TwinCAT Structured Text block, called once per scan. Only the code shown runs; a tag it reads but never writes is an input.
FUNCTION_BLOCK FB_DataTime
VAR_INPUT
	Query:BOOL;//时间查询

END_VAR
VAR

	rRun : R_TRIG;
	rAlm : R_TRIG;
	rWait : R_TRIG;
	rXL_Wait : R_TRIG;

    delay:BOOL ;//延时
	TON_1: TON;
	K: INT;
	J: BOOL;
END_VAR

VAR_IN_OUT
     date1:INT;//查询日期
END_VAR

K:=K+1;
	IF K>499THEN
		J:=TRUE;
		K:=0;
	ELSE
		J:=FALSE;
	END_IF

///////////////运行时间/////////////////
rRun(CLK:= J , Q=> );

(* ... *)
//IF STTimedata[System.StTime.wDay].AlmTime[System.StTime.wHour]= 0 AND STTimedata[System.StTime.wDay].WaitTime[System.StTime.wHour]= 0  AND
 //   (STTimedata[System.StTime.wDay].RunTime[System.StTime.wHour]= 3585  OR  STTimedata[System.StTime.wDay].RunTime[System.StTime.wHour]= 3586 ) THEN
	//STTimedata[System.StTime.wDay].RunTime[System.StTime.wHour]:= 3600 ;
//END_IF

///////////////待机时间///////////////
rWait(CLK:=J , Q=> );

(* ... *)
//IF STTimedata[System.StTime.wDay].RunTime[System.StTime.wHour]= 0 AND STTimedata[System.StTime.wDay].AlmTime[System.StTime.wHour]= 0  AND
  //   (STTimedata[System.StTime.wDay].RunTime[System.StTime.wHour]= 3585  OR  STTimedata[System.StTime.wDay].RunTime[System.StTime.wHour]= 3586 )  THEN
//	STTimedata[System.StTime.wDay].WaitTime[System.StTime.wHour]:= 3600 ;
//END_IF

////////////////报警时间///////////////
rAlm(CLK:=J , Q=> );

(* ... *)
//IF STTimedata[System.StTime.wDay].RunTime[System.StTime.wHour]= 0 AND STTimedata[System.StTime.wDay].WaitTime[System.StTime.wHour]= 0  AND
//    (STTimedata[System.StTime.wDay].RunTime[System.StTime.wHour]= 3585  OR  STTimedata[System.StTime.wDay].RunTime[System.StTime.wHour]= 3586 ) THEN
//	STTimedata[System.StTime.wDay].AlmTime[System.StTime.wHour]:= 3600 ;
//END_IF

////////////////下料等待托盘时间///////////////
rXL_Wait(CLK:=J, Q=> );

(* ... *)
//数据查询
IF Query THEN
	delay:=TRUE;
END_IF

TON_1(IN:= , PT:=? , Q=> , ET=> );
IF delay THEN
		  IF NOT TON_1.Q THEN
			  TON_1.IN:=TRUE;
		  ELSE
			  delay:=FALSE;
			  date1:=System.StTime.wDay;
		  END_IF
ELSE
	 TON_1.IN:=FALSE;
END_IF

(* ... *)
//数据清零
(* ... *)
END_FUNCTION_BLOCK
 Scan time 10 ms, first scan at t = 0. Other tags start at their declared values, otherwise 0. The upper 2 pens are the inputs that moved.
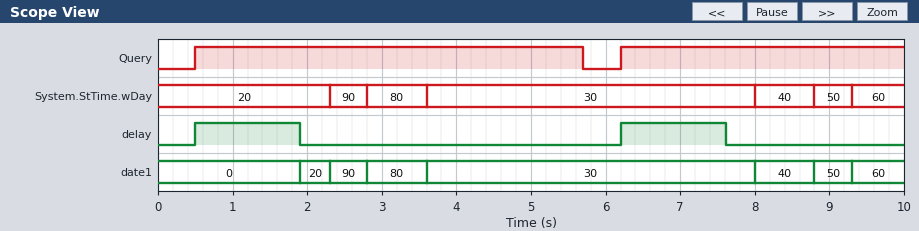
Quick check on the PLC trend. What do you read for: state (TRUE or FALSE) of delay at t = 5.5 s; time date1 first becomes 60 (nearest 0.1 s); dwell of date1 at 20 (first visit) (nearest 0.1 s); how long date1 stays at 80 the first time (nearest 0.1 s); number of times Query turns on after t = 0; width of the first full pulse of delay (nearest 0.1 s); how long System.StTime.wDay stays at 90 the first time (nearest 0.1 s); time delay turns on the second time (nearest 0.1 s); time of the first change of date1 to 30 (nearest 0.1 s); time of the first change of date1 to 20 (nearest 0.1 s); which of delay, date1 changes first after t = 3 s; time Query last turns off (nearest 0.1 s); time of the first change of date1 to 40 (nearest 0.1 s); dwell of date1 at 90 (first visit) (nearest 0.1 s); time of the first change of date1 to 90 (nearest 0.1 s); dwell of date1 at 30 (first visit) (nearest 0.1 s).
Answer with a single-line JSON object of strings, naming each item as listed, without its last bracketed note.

{"state (TRUE or FALSE) of delay at t = 5.5 s": "FALSE", "time date1 first becomes 60": "9.3 s", "dwell of date1 at 20 (first visit)": "0.4 s", "how long date1 stays at 80 the first time": "0.8 s", "number of times Query turns on after t = 0": "2", "width of the first full pulse of delay": "1.4 s", "how long System.StTime.wDay stays at 90 the first time": "0.5 s", "time delay turns on the second time": "6.2 s", "time of the first change of date1 to 30": "3.6 s", "time of the first change of date1 to 20": "1.9 s", "which of delay, date1 changes first after t = 3 s": "date1", "time Query last turns off": "5.7 s", "time of the first change of date1 to 40": "8.0 s", "dwell of date1 at 90 (first visit)": "0.5 s", "time of the first change of date1 to 90": "2.3 s", "dwell of date1 at 30 (first visit)": "4.4 s"}
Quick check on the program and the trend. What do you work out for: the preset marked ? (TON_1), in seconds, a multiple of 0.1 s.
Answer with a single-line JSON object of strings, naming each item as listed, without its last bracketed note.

{"the preset marked ? (TON_1), in seconds, a multiple of 0.1 s": "1.4 s"}
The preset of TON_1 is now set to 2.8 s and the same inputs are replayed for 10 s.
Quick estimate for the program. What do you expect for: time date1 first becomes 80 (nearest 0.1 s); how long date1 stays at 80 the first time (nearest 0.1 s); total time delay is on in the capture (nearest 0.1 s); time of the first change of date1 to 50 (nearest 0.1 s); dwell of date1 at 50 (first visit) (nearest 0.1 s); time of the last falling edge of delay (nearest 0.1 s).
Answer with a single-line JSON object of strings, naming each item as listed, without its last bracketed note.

{"time date1 first becomes 80": "3.3 s", "how long date1 stays at 80 the first time": "0.3 s", "total time delay is on in the capture": "5.6 s", "time of the first change of date1 to 50": "9.0 s", "dwell of date1 at 50 (first visit)": "0.3 s", "time of the last falling edge of delay": "9.0 s"}
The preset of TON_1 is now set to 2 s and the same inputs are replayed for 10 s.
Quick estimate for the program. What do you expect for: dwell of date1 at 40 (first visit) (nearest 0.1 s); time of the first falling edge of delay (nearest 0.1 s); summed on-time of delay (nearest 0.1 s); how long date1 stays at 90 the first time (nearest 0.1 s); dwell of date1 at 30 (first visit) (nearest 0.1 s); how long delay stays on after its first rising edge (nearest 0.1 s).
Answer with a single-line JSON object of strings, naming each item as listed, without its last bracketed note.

{"dwell of date1 at 40 (first visit)": "0.6 s", "time of the first falling edge of delay": "2.5 s", "summed on-time of delay": "4.0 s", "how long date1 stays at 90 the first time": "0.3 s", "dwell of date1 at 30 (first visit)": "4.6 s", "how long delay stays on after its first rising edge": "2.0 s"}
